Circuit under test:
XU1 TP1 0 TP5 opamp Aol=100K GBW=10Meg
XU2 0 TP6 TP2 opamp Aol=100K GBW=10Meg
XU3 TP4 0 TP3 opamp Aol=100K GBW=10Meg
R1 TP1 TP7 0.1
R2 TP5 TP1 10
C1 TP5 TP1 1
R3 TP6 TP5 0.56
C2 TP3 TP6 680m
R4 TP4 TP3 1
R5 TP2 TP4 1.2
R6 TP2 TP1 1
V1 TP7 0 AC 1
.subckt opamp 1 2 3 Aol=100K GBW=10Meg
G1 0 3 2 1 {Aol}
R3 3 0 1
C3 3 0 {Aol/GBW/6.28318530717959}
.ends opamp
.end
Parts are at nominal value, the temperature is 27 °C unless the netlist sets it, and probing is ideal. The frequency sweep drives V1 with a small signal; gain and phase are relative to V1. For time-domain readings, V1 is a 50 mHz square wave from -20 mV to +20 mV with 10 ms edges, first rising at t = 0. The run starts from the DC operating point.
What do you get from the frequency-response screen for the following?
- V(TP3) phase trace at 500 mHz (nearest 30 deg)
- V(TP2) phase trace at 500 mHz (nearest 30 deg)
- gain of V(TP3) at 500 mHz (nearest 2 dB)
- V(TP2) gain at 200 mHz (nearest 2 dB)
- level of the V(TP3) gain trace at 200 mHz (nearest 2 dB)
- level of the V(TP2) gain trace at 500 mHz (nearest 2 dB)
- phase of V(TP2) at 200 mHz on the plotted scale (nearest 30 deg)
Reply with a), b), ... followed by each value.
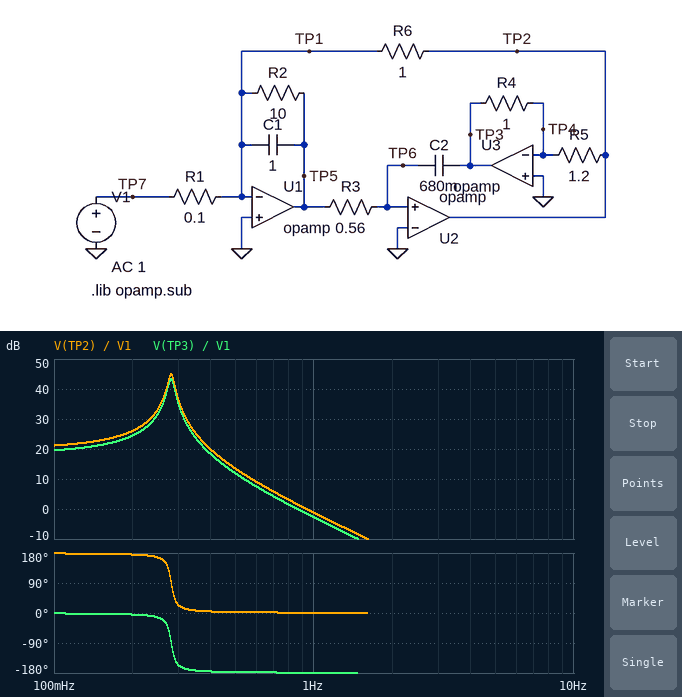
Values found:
a) -180 deg
b) 0 deg
c) 12 dB
d) 26 dB
e) 24 dB
f) 14 dB
g) 180 deg
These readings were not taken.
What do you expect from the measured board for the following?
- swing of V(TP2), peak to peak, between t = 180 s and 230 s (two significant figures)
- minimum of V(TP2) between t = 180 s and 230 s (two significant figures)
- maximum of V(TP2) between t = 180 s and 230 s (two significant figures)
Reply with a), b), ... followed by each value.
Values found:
a) 940 mV
b) -470 mV
c) 470 mV
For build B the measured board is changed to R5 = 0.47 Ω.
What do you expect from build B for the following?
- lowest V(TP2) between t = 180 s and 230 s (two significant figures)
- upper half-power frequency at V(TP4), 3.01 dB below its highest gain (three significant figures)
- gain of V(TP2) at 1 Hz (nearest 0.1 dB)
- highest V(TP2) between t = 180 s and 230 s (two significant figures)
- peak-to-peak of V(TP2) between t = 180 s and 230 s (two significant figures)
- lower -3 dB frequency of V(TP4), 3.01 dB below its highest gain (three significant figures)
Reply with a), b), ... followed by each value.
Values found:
a) -490 mV
b) 184 mHz
c) -9.8 dB
d) 490 mV
e) 980 mV
f) 168 mHz
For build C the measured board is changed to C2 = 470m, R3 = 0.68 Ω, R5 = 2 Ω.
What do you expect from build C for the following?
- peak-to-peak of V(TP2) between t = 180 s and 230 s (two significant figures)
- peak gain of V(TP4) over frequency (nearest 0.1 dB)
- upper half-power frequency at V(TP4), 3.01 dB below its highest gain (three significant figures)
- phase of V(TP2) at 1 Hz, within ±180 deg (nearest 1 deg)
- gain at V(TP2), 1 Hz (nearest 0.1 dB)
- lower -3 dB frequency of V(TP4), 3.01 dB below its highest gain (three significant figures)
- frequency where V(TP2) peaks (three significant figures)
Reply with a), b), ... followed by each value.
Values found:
a) 870 mV
b) -50.8 dB
c) 406 mHz
d) 1 deg
e) 5.5 dB
f) 390 mHz
g) 398 mHz
